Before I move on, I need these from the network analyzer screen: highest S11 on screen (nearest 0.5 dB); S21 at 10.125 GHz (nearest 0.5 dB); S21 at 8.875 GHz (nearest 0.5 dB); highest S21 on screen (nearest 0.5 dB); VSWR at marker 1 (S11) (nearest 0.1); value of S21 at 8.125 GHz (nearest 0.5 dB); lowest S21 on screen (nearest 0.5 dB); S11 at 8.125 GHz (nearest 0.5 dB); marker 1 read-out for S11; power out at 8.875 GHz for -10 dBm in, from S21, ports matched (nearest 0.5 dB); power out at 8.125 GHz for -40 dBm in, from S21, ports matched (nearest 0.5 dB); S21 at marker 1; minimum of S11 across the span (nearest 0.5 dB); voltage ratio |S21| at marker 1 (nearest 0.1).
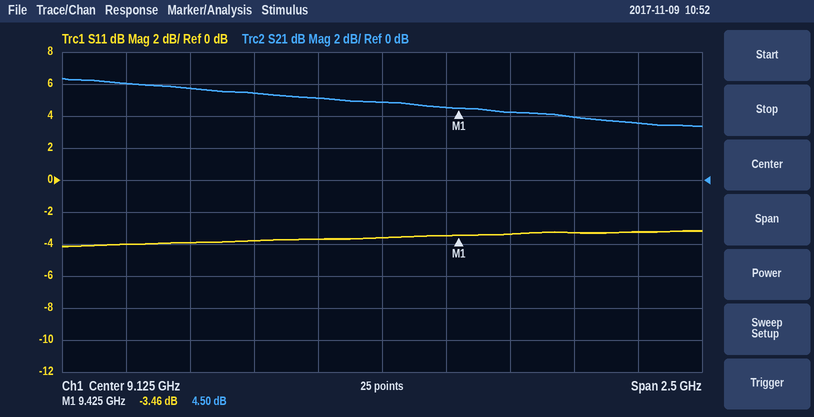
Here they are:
-3.0 dB
3.5 dB
5.0 dB
6.5 dB
5.1
6.0 dB
3.5 dB
-4.0 dB
-3.46 dB
-5.0 dBm
-34.0 dBm
4.50 dB
-4.0 dB
1.7
